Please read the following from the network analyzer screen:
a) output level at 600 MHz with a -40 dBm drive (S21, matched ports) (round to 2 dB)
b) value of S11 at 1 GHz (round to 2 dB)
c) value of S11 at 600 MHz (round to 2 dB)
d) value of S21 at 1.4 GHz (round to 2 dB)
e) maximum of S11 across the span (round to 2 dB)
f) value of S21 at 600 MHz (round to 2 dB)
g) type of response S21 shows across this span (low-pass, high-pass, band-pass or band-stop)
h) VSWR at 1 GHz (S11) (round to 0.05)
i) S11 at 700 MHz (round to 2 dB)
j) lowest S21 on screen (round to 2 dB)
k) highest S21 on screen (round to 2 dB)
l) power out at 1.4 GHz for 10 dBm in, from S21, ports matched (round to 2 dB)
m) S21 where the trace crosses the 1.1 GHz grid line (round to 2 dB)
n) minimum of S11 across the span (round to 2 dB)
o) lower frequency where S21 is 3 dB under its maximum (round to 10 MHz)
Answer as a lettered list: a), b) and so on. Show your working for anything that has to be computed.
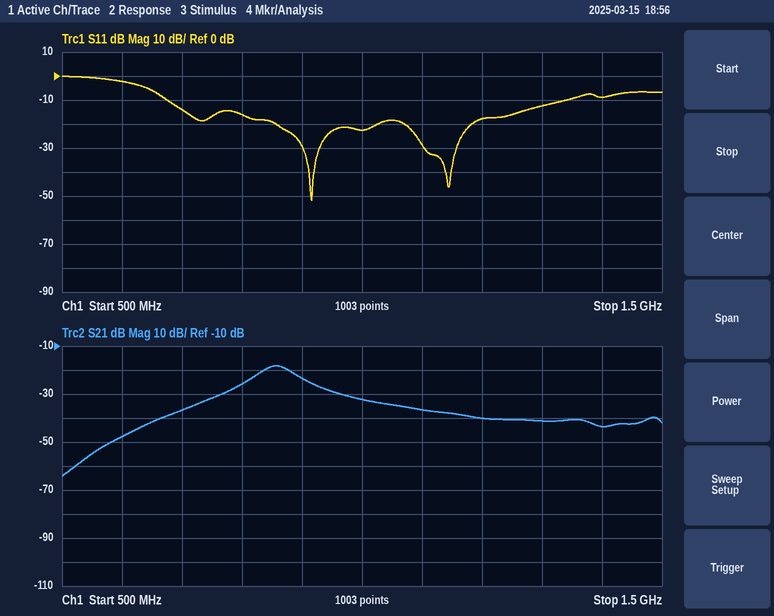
a) -40 dBm + (-48 dB) = -88 dBm
b) -22 dB
c) -2 dB
d) -44 dB
e) 0 dB
f) -48 dB
g) band-pass
h) |Γ| = 10^(-22/20) = 0.0794; VSWR = (1 + 0.0794)/(1 − 0.0794) ≈ 1.17, so 1.15 to the nearest 0.05
i) -14 dB
j) -64 dB
k) -18 dB
l) 10 dBm + (-44 dB) = -34 dBm
m) -36 dB
n) -52 dB
o) 830 MHz
